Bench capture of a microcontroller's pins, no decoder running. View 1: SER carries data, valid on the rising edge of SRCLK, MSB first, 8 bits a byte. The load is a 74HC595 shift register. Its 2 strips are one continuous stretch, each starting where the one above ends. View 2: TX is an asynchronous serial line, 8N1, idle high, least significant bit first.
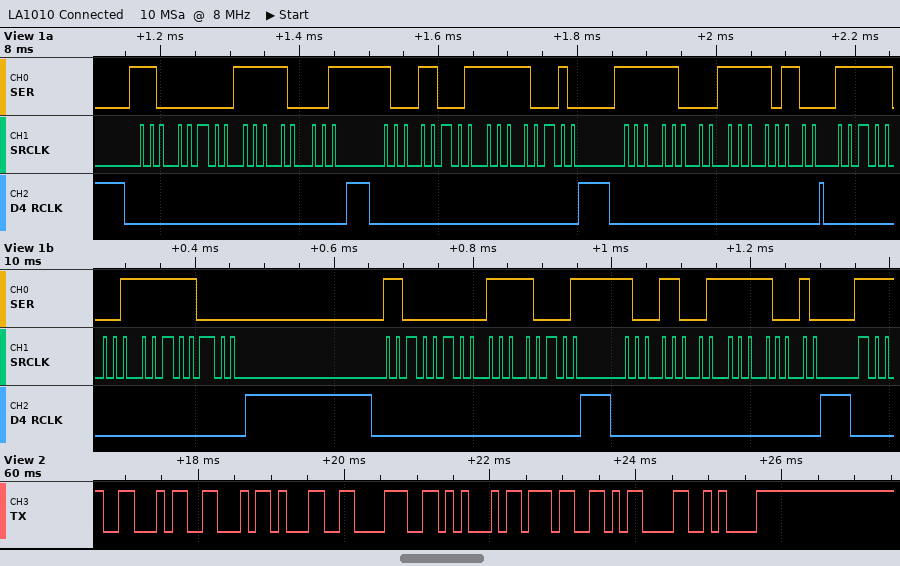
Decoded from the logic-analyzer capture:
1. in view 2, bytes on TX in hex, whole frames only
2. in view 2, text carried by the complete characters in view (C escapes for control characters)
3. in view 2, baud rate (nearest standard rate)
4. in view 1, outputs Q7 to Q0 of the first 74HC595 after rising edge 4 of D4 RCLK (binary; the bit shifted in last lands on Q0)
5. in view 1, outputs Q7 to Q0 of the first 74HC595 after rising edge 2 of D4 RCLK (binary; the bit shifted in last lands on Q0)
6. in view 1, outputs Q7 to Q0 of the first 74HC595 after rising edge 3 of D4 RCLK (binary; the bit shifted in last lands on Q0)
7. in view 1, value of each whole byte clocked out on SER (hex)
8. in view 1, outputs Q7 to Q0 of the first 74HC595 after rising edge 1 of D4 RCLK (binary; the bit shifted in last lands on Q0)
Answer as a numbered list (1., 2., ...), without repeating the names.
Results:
1. 46 46 31 38 45 37 0D 0A
2. "FF18E7\r\n"
3. 9600 baud
4. 11111000
5. 11110010
6. 11110100
7. C0 F1 99 F2 F8 F4 F9 F8 C0 F1 99 F2
8. 11110001
